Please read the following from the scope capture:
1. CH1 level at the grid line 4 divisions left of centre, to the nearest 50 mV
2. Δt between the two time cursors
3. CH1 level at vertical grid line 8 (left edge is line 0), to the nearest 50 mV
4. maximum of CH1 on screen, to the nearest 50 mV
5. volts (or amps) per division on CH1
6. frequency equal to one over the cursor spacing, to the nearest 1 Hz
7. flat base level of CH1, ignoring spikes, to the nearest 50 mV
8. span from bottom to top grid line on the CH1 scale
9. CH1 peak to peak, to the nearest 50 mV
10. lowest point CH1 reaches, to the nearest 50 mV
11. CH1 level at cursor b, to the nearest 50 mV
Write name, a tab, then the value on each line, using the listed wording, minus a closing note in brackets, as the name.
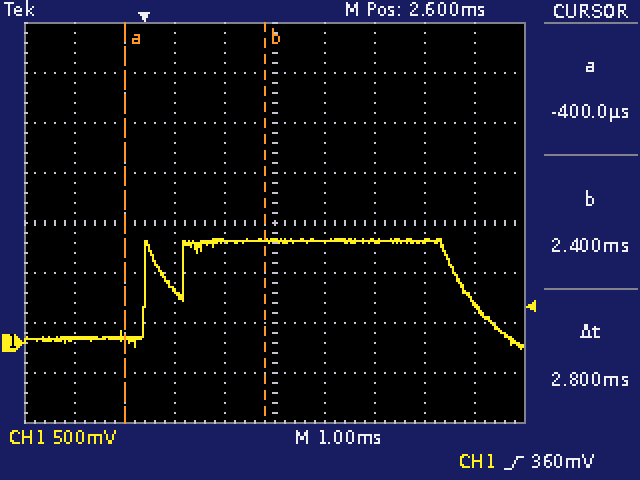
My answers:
CH1 level at the grid line 4 divisions left of centre, to the nearest 50 mV	50 mV
Δt between the two time cursors	2.8 ms
CH1 level at vertical grid line 8 (left edge is line 0), to the nearest 50 mV	1.00 V
maximum of CH1 on screen, to the nearest 50 mV	1.05 V
volts (or amps) per division on CH1	500 mV
frequency equal to one over the cursor spacing, to the nearest 1 Hz	357 Hz
flat base level of CH1, ignoring spikes, to the nearest 50 mV	50 mV
span from bottom to top grid line on the CH1 scale	4 V
CH1 peak to peak, to the nearest 50 mV	1.10 V
lowest point CH1 reaches, to the nearest 50 mV	-50 mV
CH1 level at cursor b, to the nearest 50 mV	1.00 V
